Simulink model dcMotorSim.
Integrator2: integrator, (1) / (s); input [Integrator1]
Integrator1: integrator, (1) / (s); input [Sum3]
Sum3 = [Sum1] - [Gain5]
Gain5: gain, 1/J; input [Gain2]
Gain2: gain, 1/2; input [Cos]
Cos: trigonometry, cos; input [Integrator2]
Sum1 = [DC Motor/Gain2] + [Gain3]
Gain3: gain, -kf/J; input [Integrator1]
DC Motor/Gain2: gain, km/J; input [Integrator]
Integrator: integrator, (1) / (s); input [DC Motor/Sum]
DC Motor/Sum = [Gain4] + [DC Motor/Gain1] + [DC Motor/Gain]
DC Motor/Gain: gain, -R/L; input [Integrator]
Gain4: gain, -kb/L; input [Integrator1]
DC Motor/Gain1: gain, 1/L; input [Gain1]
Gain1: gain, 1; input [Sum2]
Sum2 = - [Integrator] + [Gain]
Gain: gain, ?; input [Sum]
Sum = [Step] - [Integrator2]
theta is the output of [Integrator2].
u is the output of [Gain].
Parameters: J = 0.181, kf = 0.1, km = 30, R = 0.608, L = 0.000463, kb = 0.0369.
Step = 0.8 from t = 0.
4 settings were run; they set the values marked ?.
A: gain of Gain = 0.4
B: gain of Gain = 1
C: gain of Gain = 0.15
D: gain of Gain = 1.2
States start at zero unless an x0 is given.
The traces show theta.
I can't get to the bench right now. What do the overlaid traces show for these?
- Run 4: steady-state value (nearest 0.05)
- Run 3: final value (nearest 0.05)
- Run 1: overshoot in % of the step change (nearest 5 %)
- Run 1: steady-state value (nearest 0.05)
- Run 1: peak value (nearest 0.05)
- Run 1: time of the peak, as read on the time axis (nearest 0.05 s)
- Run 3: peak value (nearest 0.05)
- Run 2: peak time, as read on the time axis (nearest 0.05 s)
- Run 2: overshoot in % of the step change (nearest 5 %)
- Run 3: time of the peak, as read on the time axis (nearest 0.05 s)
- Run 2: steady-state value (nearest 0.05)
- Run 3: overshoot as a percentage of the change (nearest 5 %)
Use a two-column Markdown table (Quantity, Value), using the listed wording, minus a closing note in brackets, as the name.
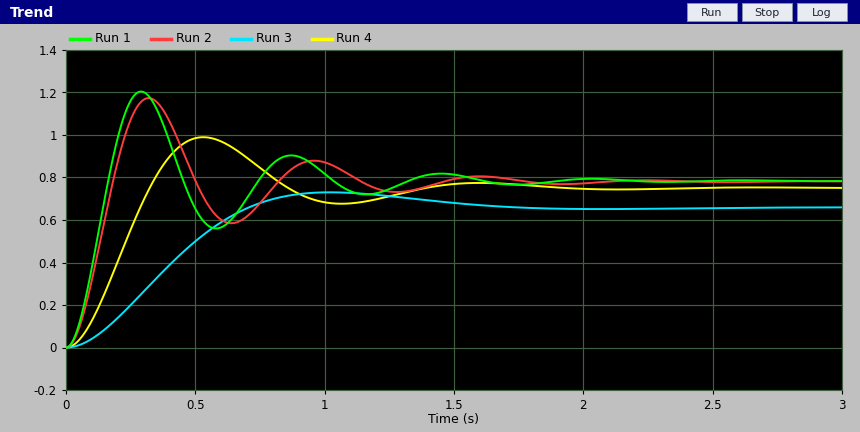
| Quantity | Value |
|---|---|
| Run 4: steady-state value | 0.75 |
| Run 3: final value | 0.65 |
| Run 1: overshoot in % of the step change | 55 % |
| Run 1: steady-state value | 0.80 |
| Run 1: peak value | 1.20 |
| Run 1: time of the peak, as read on the time axis | 0.30 s |
| Run 3: peak value | 0.75 |
| Run 2: peak time, as read on the time axis | 0.30 s |
| Run 2: overshoot in % of the step change | 50 % |
| Run 3: time of the peak, as read on the time axis | 1.00 s |
| Run 2: steady-state value | 0.80 |
| Run 3: overshoot as a percentage of the change | 10 % |
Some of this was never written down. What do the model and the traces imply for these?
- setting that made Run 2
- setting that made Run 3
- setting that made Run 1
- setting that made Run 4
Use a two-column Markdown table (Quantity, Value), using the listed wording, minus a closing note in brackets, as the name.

| Quantity | Value |
|---|---|
| setting that made Run 2 | B |
| setting that made Run 3 | C |
| setting that made Run 1 | D |
| setting that made Run 4 | A |
